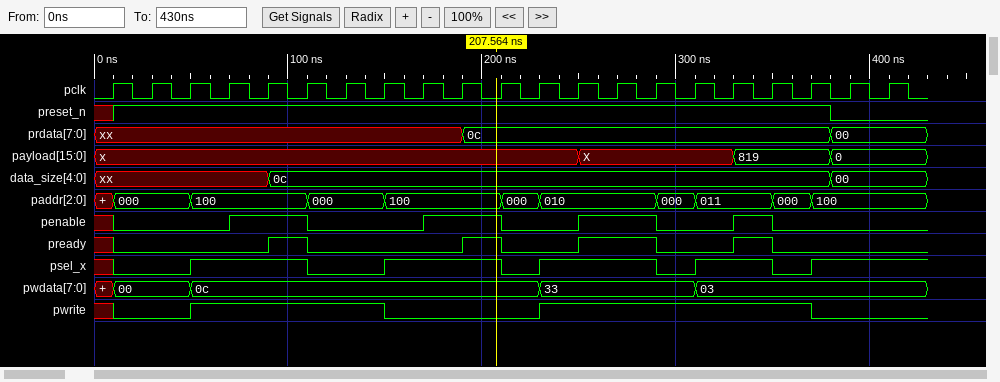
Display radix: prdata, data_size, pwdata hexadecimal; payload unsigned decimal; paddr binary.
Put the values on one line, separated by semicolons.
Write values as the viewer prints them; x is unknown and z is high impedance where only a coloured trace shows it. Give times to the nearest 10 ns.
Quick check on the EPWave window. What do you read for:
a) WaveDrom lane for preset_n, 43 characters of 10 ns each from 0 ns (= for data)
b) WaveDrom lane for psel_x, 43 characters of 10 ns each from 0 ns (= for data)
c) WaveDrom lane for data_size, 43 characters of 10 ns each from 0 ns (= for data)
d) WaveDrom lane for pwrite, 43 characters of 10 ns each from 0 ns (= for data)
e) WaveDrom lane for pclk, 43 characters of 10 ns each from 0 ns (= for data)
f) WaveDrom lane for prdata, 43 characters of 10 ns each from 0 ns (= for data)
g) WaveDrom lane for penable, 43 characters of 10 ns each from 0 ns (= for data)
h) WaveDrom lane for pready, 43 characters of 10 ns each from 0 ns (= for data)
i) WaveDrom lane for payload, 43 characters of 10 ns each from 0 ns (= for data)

{name: 'preset_n', wave: 'x1....................................0....'}; {name: 'psel_x', wave: 'x0...1.....0...1.....0.1.....0.1...0.1.....'}; {name: 'data_size', wave: 'x........=............................=....', data: '0c 00'}; {name: 'pwrite', wave: 'x0...1.........0.......1.............0.....'}; {name: 'pclk', wave: '0101010101010101010101010101010101010101010'}; {name: 'prdata', wave: 'x..................=..................=....', data: '0c 00'}; {name: 'penable', wave: 'x0.....1...0.....1...0...1...0...1.0.......'}; {name: 'pready', wave: 'x0.......1.0.......1.0...1...0...1.0.......'}; {name: 'payload', wave: 'x........................=.......=....=....', data: 'X 819 0'}
